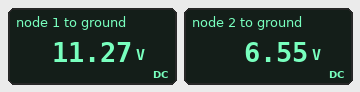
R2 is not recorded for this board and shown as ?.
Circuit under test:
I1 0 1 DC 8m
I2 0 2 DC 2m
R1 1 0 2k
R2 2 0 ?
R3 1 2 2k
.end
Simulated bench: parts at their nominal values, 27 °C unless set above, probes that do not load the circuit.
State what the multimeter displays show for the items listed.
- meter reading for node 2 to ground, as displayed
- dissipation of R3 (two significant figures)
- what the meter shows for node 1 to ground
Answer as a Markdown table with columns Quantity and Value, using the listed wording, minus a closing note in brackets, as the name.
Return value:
| Quantity | Value |
|---|---|
| meter reading for node 2 to ground, as displayed | 6.55 V |
| dissipation of R3 | 11 mW |
| what the meter shows for node 1 to ground | 11.27 V |
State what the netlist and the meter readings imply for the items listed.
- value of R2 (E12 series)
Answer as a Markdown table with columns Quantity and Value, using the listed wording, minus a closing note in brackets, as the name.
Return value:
| Quantity | Value |
|---|---|
| value of R2 | 1.5 kΩ |
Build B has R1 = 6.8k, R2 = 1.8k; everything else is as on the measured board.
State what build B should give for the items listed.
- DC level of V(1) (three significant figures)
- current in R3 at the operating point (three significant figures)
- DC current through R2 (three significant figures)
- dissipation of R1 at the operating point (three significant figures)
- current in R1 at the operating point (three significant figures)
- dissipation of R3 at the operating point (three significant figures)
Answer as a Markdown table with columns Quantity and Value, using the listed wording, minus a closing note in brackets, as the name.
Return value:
| Quantity | Value |
|---|---|
| DC level of V(1) | 21.8 V |
| current in R3 at the operating point | 4.79 mA |
| DC current through R2 | 6.79 mA |
| dissipation of R1 at the operating point | 70.0 mW |
| current in R1 at the operating point | 3.21 mA |
| dissipation of R3 at the operating point | 45.9 mW |
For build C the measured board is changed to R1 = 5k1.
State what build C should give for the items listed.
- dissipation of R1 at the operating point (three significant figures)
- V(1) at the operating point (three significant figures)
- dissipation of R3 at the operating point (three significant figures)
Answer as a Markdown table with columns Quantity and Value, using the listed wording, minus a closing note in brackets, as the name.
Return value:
| Quantity | Value |
|---|---|
| dissipation of R1 at the operating point | 66.3 mW |
| V(1) at the operating point | 18.4 V |
| dissipation of R3 at the operating point | 38.6 mW |
